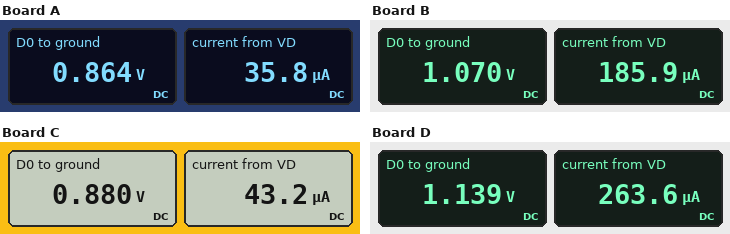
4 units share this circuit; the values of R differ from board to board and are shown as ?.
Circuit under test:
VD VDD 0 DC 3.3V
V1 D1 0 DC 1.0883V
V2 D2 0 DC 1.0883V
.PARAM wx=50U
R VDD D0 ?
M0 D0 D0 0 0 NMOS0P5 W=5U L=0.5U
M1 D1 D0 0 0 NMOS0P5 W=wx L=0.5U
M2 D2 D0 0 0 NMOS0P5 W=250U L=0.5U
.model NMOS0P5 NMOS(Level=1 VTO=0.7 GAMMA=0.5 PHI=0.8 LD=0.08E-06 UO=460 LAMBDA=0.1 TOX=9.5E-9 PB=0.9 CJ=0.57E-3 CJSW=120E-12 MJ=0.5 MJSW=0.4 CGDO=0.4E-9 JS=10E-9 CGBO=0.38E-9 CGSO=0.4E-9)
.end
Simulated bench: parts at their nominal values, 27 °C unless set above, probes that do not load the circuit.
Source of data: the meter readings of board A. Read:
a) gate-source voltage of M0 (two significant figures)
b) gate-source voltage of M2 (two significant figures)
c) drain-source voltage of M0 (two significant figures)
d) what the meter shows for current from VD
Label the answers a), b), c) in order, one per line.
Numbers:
a) 860 mV
b) 860 mV
c) 860 mV
d) 35.8 µA
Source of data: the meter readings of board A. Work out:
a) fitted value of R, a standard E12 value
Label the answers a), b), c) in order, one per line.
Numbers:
a) 68 kΩ
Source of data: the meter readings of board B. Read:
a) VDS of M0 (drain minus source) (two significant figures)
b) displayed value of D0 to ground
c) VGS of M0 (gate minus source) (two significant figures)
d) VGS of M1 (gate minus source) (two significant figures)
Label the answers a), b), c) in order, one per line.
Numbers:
a) 1.1 V
b) 1.070 V
c) 1.1 V
d) 1.1 V
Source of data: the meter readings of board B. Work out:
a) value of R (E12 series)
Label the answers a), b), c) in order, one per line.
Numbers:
a) 12 kΩ
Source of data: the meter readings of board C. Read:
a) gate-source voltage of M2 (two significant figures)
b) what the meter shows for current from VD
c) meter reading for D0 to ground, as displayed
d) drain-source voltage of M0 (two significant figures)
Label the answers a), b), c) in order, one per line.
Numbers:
a) 880 mV
b) 43.2 µA
c) 0.880 V
d) 880 mV
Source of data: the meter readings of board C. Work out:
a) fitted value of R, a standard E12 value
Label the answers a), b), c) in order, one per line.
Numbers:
a) 56 kΩ
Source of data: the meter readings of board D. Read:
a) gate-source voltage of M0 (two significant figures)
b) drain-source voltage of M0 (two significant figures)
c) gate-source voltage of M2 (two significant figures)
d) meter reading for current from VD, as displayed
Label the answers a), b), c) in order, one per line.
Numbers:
a) 1.1 V
b) 1.1 V
c) 1.1 V
d) 263.6 µA
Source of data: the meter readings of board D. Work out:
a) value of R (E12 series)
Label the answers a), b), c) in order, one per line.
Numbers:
a) 8.2 kΩ
